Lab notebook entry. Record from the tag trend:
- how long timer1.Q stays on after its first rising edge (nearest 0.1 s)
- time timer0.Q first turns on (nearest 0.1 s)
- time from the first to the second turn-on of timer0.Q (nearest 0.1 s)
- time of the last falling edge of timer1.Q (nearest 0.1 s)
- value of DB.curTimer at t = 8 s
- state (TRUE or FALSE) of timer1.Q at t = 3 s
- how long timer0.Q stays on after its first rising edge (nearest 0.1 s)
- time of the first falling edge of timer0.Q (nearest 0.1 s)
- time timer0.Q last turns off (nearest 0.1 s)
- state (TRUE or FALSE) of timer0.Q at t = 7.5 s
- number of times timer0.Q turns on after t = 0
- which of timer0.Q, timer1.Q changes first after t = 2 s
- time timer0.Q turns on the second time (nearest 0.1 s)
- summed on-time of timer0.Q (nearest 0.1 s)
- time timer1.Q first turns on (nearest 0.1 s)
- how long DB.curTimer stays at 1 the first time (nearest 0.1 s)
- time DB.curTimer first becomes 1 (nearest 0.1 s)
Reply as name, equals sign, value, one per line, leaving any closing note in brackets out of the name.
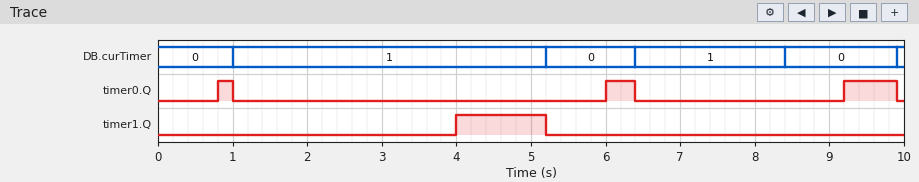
how long timer1.Q stays on after its first rising edge = 1.2 s
time timer0.Q first turns on = 0.8 s
time from the first to the second turn-on of timer0.Q = 5.2 s
time of the last falling edge of timer1.Q = 5.2 s
value of DB.curTimer at t = 8 s = 1
state (TRUE or FALSE) of timer1.Q at t = 3 s = FALSE
how long timer0.Q stays on after its first rising edge = 0.2 s
time of the first falling edge of timer0.Q = 1.0 s
time timer0.Q last turns off = 9.9 s
state (TRUE or FALSE) of timer0.Q at t = 7.5 s = FALSE
number of times timer0.Q turns on after t = 0 = 3
which of timer0.Q, timer1.Q changes first after t = 2 s = timer1.Q
time timer0.Q turns on the second time = 6.0 s
summed on-time of timer0.Q = 1.3 s
time timer1.Q first turns on = 4.0 s
how long DB.curTimer stays at 1 the first time = 4.2 s
time DB.curTimer first becomes 1 = 1.0 s
